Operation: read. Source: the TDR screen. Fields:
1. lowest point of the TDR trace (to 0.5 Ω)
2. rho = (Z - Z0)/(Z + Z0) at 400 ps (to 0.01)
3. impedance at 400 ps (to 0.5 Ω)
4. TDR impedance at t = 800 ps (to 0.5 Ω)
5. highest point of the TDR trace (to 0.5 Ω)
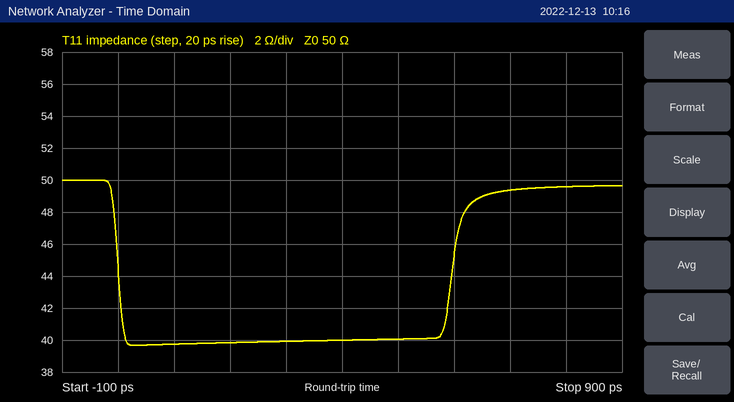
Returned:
39.5 Ω
-0.11
40.0 Ω
49.5 Ω
50.0 Ω
